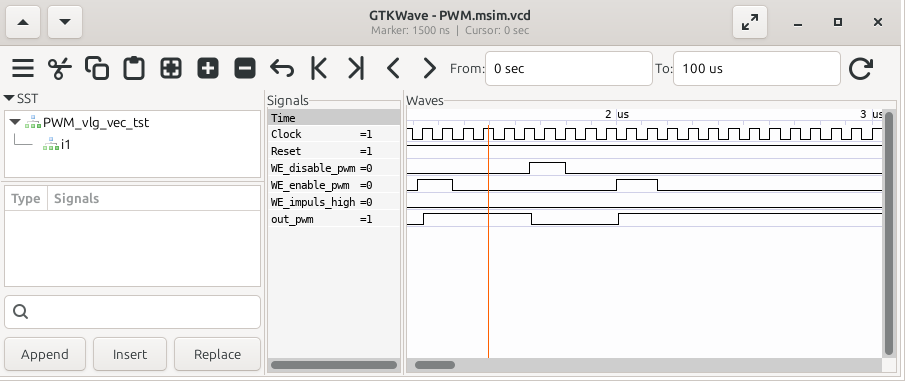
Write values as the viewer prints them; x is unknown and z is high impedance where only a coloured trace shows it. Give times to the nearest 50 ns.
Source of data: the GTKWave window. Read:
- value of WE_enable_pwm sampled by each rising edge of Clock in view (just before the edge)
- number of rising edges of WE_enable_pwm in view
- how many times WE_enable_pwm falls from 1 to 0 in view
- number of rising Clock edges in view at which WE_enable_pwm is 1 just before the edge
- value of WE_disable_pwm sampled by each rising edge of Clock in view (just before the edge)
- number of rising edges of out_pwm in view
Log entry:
1 1 0 0 0 0 0 0 0 0 1 1 0 0 0 0 0 0 0 0 0 0 0
2
2
4
0 0 0 0 0 0 1 1 0 0 0 0 0 0 0 0 0 0 0 0 0 0 0
2
